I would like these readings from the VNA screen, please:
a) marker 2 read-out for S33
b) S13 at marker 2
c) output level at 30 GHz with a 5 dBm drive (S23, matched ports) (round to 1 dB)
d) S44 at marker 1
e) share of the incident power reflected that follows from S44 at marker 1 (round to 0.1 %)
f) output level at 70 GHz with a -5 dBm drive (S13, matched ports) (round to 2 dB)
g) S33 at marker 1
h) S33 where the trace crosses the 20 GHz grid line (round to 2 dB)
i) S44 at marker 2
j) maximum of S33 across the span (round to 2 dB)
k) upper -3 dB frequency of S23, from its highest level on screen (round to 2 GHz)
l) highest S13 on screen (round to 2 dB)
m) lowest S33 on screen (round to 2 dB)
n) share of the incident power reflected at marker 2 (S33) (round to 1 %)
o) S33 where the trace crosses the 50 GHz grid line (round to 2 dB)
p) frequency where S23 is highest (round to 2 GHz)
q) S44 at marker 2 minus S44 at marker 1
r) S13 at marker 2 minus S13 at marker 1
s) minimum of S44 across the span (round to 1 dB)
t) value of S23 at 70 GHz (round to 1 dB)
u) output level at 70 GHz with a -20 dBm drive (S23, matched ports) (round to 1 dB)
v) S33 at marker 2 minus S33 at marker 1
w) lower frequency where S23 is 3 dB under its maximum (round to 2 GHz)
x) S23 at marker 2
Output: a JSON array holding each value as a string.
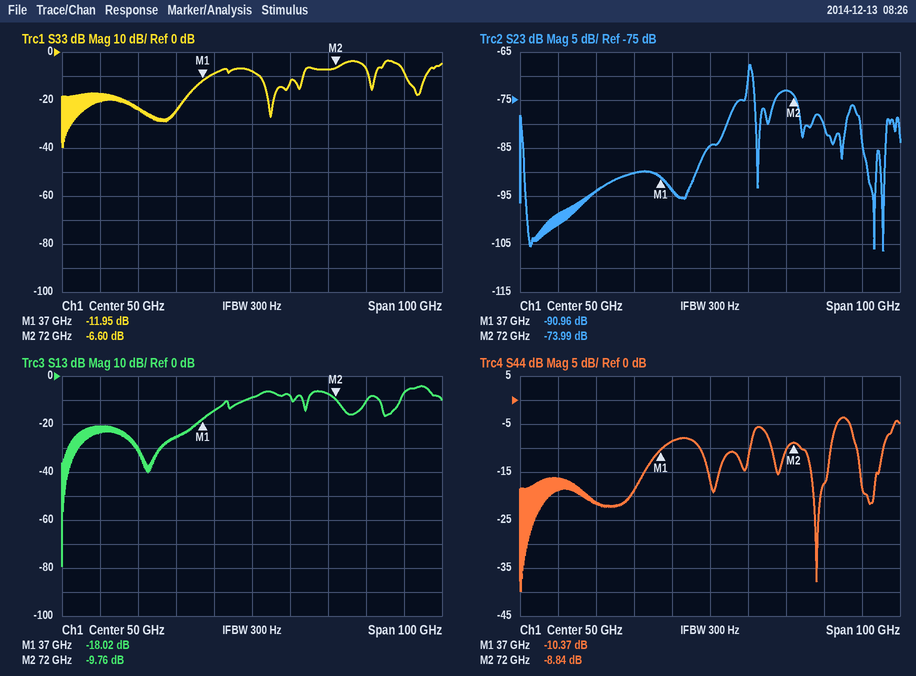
["-6.60 dB", "-9.76 dB", "-85 dBm", "-10.37 dB", "9.2 %", "-12 dBm", "-11.95 dB", "-24 dB", "-8.84 dB", "-4 dB", "62 GHz", "-4 dB", "-40 dB", "22 %", "-8 dB", "60 GHz", "1.53 dB", "8.26 dB", "-40 dB", "-73 dB", "-93 dBm", "5.35 dB", "60 GHz", "-73.99 dB"]
